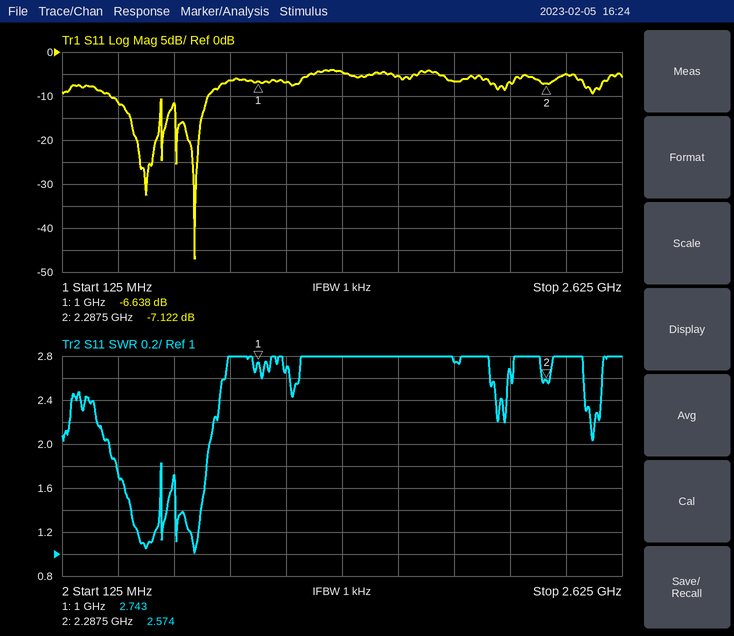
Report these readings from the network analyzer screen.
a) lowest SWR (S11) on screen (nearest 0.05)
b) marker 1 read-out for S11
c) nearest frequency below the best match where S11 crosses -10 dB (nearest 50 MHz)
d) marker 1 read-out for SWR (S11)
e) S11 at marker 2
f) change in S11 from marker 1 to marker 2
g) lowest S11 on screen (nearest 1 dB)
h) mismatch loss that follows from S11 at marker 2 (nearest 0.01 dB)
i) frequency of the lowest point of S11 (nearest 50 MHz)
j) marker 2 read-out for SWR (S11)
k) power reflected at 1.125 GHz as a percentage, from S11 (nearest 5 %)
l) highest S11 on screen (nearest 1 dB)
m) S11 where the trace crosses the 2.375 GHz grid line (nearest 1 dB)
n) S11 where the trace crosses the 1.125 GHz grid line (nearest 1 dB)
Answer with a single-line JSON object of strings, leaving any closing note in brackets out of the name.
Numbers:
{"lowest SWR (S11) on screen": "1.00", "marker 1 read-out for S11": "-6.638 dB", "nearest frequency below the best match where S11 crosses -10 dB": "350 MHz", "marker 1 read-out for SWR": "2.743", "S11 at marker 2": "-7.122 dB", "change in S11 from marker 1 to marker 2": "-0.484 dB", "lowest S11 on screen": "-47 dB", "mismatch loss that follows from S11 at marker 2": "0.94 dB", "frequency of the lowest point of S11": "700 MHz", "marker 2 read-out for SWR": "2.574", "power reflected at 1.125 GHz as a percentage, from S11": "20 %", "highest S11 on screen": "-4 dB", "S11 where the trace crosses the 2.375 GHz grid line": "-5 dB", "S11 where the trace crosses the 1.125 GHz grid line": "-7 dB"}
